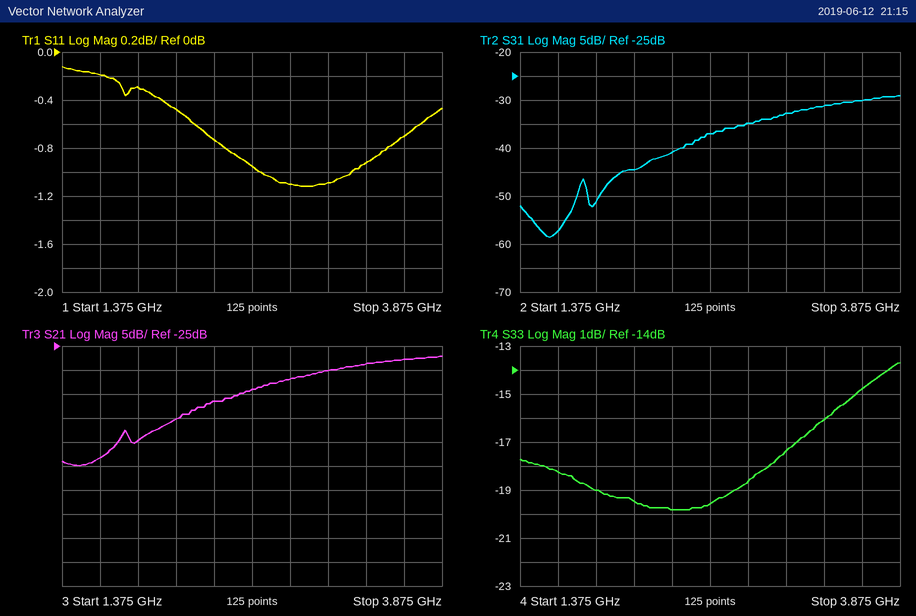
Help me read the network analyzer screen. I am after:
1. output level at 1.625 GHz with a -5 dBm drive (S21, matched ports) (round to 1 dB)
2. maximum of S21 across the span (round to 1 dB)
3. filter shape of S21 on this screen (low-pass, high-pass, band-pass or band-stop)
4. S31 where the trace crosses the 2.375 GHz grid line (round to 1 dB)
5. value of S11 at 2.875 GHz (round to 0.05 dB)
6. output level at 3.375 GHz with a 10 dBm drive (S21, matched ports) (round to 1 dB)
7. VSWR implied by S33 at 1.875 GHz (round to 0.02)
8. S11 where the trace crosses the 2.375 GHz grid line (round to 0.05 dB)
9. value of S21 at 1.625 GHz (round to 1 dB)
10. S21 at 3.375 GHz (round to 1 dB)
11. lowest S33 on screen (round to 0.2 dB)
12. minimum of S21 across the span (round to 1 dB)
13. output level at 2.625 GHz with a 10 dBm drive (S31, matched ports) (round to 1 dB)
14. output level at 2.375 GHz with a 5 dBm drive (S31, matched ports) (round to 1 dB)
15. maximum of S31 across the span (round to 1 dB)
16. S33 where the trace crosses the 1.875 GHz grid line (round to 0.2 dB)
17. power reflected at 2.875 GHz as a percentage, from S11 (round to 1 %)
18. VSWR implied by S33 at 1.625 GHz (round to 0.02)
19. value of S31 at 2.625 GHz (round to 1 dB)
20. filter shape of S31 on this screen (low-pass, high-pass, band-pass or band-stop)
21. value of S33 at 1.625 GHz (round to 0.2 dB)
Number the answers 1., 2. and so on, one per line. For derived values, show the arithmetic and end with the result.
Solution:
1. -5 dBm + (-48 dB) = -53 dBm
2. -27 dB
3. high-pass
4. -41 dB
5. -1.10 dB
6. 10 dBm + (-29 dB) = -19 dBm
7. |Γ| = 10^(-19/20) = 0.1122; VSWR = (1 + 0.1122)/(1 − 0.1122) ≈ 1.25, so 1.26 to the nearest 0.02
8. -0.75 dB
9. -48 dB
10. -29 dB
11. -19.8 dB
12. -50 dB
13. 10 dBm + (-37 dB) = -27 dBm
14. 5 dBm + (-41 dB) = -36 dBm
15. -29 dB
16. -19.0 dB
17. 10^(-1.1/10) ≈ 78 %
18. |Γ| = 10^(-18.2/20) = 0.1230; VSWR = (1 + 0.1230)/(1 − 0.1230) ≈ 1.28
19. -37 dB
20. high-pass
21. -18.2 dB
